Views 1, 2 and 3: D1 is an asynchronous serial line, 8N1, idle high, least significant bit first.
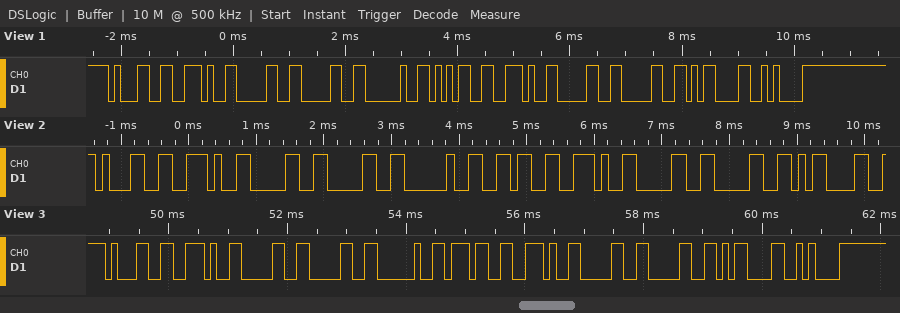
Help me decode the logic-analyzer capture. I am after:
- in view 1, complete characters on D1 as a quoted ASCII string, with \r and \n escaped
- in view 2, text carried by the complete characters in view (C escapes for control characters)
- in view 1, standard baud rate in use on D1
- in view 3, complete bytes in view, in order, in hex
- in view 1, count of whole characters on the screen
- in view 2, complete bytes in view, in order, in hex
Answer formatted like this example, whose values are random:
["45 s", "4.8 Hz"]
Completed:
["\"1.00 5.00\\r\\n\"", "\"1.00 6.00\\r\"", "9600 baud", "31 2E 30 30 20 37 2E 30 30 0D 0A", "11", "31 2E 30 30 20 36 2E 30 30 0D"]
